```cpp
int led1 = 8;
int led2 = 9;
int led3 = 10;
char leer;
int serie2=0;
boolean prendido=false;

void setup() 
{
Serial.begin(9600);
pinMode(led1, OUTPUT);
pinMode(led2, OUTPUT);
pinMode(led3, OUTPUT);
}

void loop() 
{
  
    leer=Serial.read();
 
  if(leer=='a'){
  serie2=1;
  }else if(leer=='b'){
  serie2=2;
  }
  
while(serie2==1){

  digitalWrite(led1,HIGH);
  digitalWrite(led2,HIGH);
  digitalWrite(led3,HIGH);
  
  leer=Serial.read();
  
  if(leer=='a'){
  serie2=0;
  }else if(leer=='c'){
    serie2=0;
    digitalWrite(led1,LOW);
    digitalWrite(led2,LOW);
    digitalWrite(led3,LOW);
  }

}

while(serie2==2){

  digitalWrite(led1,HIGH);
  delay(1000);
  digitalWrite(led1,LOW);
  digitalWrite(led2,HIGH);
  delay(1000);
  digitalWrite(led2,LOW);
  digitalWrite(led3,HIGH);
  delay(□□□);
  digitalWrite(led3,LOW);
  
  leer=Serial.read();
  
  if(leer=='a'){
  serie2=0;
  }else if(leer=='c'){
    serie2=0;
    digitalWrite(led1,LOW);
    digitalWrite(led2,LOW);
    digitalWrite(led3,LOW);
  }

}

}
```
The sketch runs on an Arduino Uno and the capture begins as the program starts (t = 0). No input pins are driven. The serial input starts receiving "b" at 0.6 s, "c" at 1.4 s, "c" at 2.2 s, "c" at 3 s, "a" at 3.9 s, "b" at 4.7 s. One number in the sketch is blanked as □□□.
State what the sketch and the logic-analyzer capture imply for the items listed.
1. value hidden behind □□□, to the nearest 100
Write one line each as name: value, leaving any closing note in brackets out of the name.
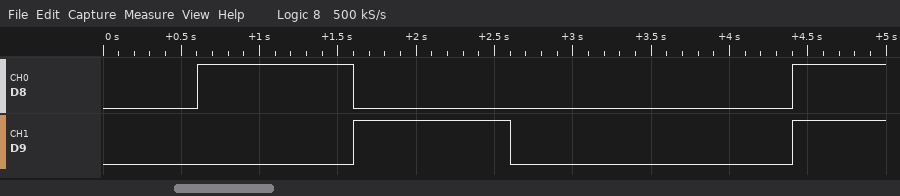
value hidden behind □□□, to the nearest 100: 1800
